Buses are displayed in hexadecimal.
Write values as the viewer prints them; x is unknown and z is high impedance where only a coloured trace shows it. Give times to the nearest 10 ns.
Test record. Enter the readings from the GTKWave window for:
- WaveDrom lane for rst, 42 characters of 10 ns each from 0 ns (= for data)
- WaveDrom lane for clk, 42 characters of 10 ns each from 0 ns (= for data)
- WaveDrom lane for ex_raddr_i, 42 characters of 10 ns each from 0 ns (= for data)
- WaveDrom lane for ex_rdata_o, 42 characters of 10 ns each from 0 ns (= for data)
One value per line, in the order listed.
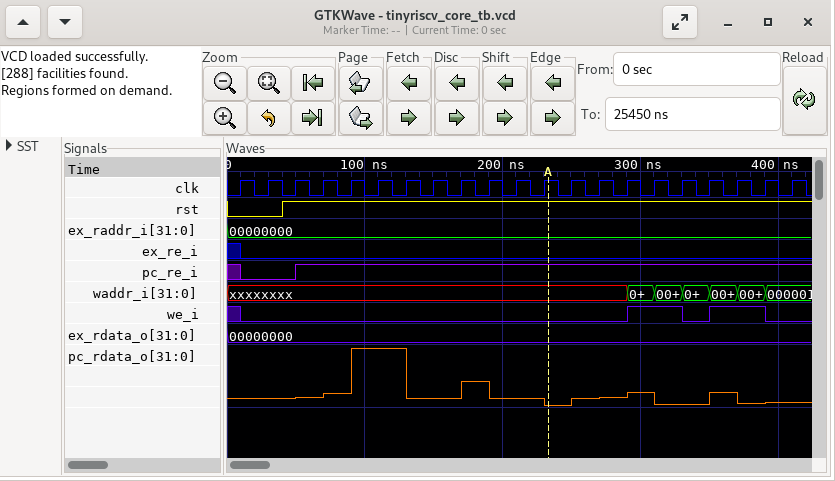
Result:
{name: 'rst', wave: '0...1.....................................'}
{name: 'clk', wave: '010101010101010101010101010101010101010101'}
{name: 'ex_raddr_i', wave: '=.........................................', data: '00000000'}
{name: 'ex_rdata_o', wave: '=.........................................', data: '00000000'}
